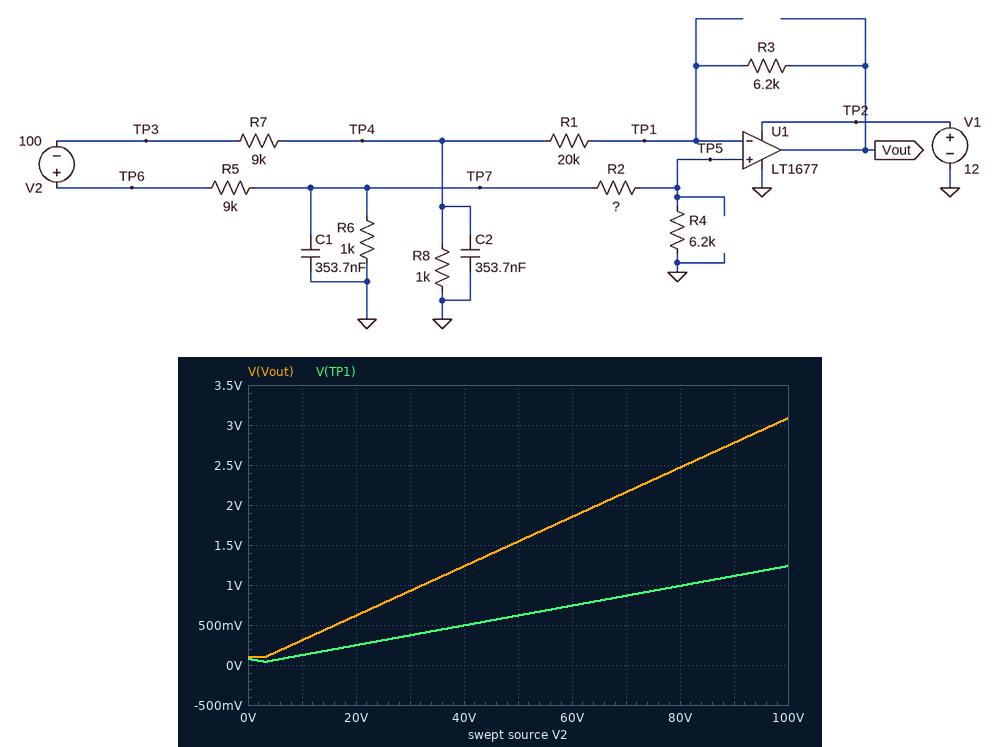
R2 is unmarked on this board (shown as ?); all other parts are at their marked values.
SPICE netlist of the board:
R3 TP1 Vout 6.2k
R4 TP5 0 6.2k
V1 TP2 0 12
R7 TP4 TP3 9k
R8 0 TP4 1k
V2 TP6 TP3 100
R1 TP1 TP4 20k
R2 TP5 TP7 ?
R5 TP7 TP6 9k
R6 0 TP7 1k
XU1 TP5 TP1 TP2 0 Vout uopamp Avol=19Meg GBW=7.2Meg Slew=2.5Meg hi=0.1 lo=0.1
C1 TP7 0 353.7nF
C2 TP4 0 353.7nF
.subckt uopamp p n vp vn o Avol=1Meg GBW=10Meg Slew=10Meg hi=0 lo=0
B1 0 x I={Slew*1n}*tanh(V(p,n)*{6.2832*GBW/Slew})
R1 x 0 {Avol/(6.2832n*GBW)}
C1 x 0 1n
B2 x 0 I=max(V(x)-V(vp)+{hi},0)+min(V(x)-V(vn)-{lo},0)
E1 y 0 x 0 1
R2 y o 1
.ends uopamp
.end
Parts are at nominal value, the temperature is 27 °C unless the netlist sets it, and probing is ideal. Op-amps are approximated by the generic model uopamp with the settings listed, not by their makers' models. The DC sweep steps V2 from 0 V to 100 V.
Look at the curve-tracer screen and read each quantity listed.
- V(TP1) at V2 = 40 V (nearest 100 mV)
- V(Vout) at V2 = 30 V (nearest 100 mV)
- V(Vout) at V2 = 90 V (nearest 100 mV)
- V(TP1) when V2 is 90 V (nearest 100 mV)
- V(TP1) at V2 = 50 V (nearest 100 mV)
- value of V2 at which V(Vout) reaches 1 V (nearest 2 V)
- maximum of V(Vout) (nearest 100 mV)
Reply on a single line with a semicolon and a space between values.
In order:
500 mV; 900 mV; 2.8 V; 1.1 V; 600 mV; 32 V; 3.1 V
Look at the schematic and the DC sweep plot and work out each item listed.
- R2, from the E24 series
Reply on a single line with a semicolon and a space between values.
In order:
18 kΩ
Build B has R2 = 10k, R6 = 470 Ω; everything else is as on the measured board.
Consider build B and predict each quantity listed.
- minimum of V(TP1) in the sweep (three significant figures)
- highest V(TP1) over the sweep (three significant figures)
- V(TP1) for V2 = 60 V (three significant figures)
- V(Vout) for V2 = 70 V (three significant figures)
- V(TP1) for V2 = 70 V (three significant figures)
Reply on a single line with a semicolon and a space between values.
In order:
33.8 mV; 901 mV; 541 mV; 1.88 V; 631 mV
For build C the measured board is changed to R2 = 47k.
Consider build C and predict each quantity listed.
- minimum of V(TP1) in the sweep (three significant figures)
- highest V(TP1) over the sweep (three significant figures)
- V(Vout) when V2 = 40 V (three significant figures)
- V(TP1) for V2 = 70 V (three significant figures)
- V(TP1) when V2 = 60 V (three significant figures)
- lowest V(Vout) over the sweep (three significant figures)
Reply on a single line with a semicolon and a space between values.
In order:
25.8 mV; 574 mV; 890 mV; 402 mV; 344 mV; 97.8 mV
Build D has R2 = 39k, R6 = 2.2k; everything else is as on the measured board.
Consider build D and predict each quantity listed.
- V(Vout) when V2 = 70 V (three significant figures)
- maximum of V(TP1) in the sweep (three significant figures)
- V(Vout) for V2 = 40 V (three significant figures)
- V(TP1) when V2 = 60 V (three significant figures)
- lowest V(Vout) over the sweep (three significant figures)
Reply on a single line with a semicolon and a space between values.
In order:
2.22 V; 1.37 V; 1.27 V; 821 mV; 97.8 mV
